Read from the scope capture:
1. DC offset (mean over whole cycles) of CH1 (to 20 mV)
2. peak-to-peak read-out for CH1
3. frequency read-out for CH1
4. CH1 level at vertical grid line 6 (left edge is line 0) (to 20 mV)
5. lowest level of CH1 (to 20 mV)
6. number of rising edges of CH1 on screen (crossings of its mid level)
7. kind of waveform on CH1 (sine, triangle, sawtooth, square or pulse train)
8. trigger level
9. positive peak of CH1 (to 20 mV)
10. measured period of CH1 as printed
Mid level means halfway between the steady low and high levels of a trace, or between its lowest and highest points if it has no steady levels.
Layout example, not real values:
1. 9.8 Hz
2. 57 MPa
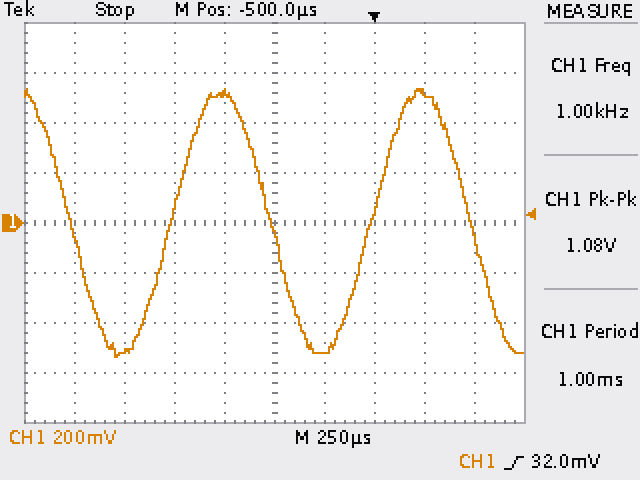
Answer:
1. 0 mV
2. 1.08 V
3. 1.00 kHz
4. -520 mV
5. -540 mV
6. 2
7. sine
8. 32.0 mV
9. 540 mV
10. 1.00 ms
